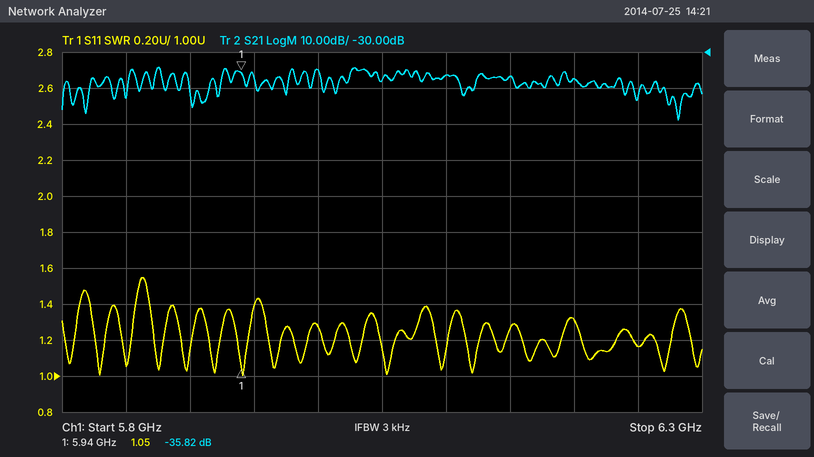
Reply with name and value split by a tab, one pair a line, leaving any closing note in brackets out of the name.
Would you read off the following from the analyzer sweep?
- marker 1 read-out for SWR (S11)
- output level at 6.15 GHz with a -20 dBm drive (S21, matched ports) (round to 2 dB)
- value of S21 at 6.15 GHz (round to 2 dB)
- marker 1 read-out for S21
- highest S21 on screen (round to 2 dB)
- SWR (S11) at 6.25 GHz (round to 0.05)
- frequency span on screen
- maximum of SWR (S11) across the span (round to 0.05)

marker 1 read-out for SWR	1.05
output level at 6.15 GHz with a -20 dBm drive (S21, matched ports)	-56 dBm
value of S21 at 6.15 GHz	-36 dB
marker 1 read-out for S21	-35.82 dB
highest S21 on screen	-34 dB
SWR (S11) at 6.25 GHz	1.15
frequency span on screen	500 MHz
maximum of SWR (S11) across the span	1.55
